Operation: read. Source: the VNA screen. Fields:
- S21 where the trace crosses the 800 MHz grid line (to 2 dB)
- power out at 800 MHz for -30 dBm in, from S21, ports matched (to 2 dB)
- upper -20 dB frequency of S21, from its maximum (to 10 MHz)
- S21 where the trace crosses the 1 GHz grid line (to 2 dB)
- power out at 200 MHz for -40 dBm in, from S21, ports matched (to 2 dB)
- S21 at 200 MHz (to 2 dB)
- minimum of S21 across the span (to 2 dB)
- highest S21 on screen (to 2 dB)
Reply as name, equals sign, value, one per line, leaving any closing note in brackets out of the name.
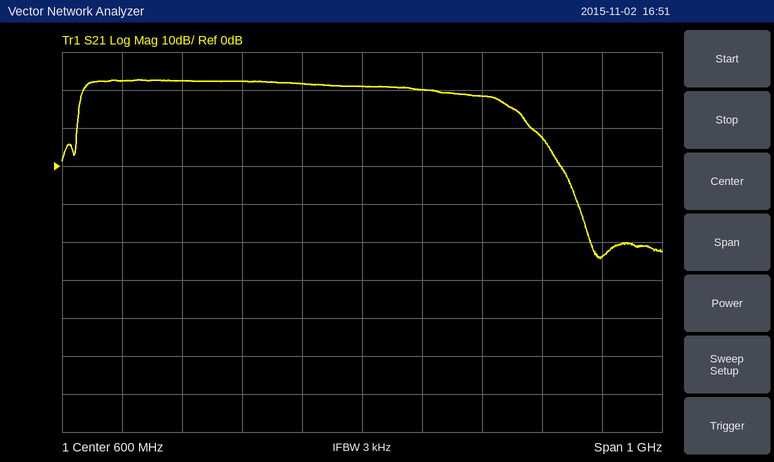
S21 where the trace crosses the 800 MHz grid line = 18 dB
power out at 800 MHz for -30 dBm in, from S21, ports matched = -12 dBm
upper -20 dB frequency of S21, from its maximum = 920 MHz
S21 where the trace crosses the 1 GHz grid line = -24 dB
power out at 200 MHz for -40 dBm in, from S21, ports matched = -18 dBm
S21 at 200 MHz = 22 dB
minimum of S21 across the span = -24 dB
highest S21 on screen = 22 dB
